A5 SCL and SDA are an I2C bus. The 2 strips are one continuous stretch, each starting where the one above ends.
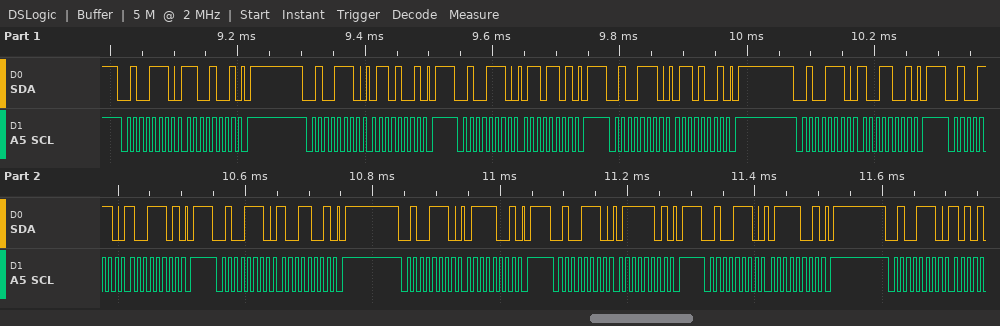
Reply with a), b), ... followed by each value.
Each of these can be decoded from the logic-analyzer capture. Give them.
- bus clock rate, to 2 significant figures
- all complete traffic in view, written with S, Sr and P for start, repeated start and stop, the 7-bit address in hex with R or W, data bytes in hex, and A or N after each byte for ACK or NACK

a) 100 kHz
b) S 27W A C9 A P S 27W A 69 A P S 27W A 6D A P S 27W A 69 A P S 27W A 99 A P S 27W A 9D A P S 27W A 99 A P S 27W A 79 A P S 27W A 7D A P S 27W A 79 A P S 27W A
